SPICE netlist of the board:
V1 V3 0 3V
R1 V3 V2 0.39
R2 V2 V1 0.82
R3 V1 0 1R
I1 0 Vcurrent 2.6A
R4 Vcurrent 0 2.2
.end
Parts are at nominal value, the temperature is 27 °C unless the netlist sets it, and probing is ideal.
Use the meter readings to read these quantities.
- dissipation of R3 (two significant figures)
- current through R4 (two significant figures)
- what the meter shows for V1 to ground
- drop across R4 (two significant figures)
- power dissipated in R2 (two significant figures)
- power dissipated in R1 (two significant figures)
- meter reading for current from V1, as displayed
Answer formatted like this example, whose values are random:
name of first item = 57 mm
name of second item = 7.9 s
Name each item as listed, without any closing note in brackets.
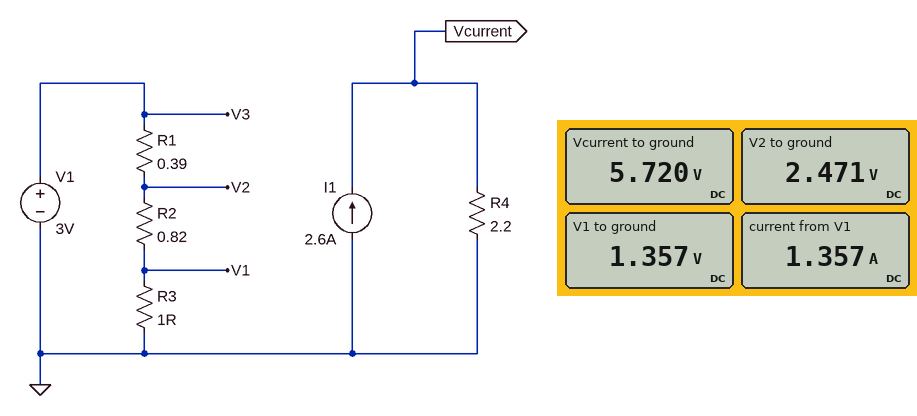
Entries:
dissipation of R3 = 1.8 W
current through R4 = 2.6 A
what the meter shows for V1 to ground = 1.357 V
drop across R4 = 5.7 V
power dissipated in R2 = 1.5 W
power dissipated in R1 = 720 mW
meter reading for current from V1, as displayed = 1.357 A
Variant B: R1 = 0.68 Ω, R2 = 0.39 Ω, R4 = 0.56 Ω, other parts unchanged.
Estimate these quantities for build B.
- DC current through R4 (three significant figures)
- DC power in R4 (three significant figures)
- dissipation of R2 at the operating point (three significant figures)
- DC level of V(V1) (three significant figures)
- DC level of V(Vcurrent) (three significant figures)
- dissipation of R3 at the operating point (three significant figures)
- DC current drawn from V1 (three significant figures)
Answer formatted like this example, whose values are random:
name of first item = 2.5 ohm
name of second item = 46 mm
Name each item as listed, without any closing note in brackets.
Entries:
DC current through R4 = 2.60 A
DC power in R4 = 3.79 W
dissipation of R2 at the operating point = 819 mW
DC level of V(V1) = 1.45 V
DC level of V(Vcurrent) = 1.46 V
dissipation of R3 at the operating point = 2.10 W
DC current drawn from V1 = 1.45 A
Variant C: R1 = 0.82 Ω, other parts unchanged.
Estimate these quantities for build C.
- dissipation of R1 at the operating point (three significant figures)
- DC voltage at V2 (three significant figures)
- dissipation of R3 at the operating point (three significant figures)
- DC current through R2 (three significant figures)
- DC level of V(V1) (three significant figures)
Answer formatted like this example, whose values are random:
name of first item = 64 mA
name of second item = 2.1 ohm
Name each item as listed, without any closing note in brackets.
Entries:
dissipation of R1 at the operating point = 1.06 W
DC voltage at V2 = 2.07 V
dissipation of R3 at the operating point = 1.29 W
DC current through R2 = 1.14 A
DC level of V(V1) = 1.14 V
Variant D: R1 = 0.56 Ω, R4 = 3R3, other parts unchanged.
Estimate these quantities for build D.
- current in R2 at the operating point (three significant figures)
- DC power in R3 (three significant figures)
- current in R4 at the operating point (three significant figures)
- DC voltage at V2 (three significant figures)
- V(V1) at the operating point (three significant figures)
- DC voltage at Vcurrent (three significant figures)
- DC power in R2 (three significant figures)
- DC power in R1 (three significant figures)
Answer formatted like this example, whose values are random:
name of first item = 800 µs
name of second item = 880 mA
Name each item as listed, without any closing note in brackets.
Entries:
current in R2 at the operating point = 1.26 A
DC power in R3 = 1.59 W
current in R4 at the operating point = 2.60 A
DC voltage at V2 = 2.29 V
V(V1) at the operating point = 1.26 V
DC voltage at Vcurrent = 8.58 V
DC power in R2 = 1.30 W
DC power in R1 = 890 mW
